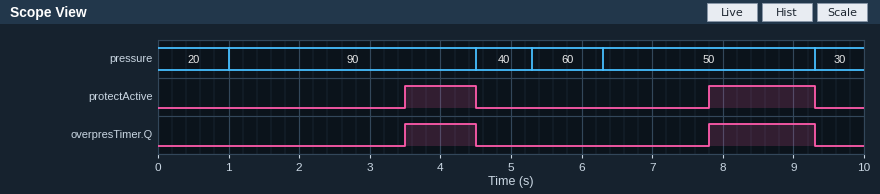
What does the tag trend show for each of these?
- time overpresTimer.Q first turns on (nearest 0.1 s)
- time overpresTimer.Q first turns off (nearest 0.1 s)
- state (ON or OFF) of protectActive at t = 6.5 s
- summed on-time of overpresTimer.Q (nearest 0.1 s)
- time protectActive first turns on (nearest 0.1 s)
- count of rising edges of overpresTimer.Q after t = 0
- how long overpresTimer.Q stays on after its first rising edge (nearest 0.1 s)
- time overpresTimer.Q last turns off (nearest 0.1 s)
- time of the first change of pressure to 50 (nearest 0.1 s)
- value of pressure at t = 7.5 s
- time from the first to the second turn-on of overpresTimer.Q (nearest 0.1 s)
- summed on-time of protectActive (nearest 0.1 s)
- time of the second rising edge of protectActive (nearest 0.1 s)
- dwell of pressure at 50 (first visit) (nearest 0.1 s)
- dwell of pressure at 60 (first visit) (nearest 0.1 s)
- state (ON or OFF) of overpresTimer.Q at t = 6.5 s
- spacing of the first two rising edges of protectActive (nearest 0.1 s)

3.5 s
4.5 s
OFF
2.5 s
3.5 s
2
1.0 s
9.3 s
6.3 s
50
4.3 s
2.5 s
7.8 s
3.0 s
1.0 s
OFF
4.3 s
